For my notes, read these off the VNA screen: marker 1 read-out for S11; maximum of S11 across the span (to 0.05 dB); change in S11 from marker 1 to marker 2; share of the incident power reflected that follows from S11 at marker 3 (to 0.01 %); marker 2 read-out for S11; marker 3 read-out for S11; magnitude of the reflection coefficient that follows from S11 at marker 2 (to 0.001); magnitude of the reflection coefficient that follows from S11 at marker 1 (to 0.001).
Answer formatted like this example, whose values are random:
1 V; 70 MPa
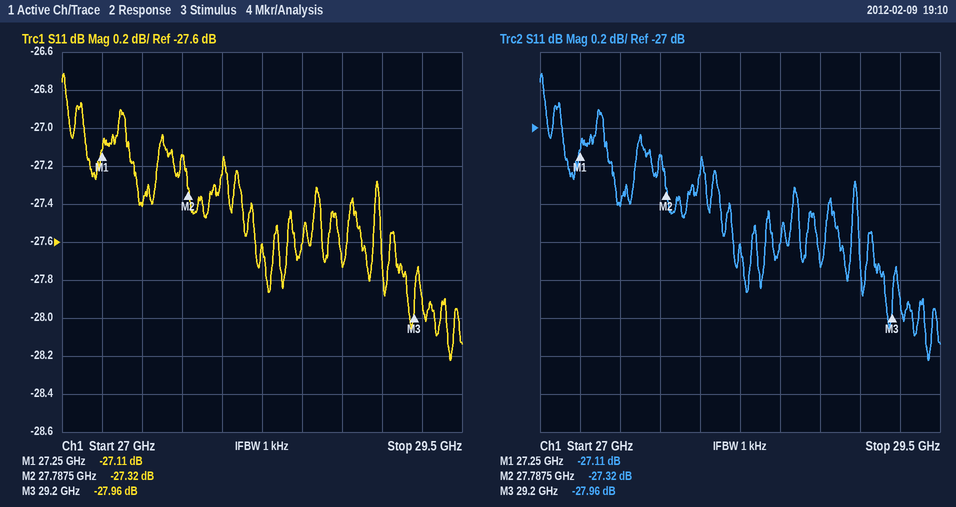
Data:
-27.11 dB; -26.70 dB; -0.21 dB; 0.16 %; -27.32 dB; -27.96 dB; 0.043; 0.044
